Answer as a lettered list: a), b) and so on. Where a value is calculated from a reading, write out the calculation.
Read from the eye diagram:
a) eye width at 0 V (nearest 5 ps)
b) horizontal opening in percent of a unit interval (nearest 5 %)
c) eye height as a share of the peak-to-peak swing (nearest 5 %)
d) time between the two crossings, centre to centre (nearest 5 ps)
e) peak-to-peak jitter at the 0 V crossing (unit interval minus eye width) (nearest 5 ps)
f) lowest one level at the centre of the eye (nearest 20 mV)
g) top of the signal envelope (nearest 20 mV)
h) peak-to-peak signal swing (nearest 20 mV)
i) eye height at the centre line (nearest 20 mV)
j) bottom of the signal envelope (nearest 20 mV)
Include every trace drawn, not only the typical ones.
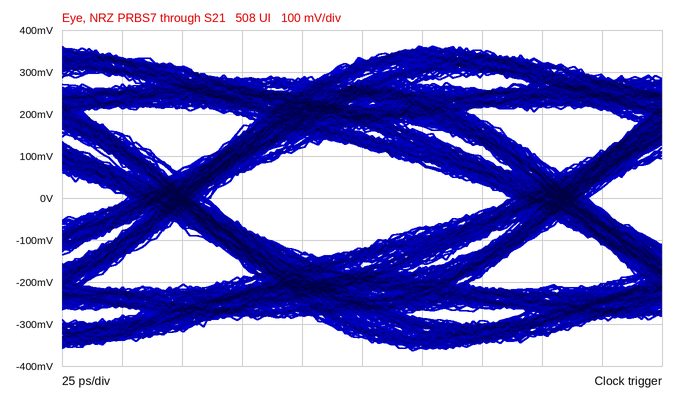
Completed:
a) 125 ps
b) 125 ps / 160 ps ≈ 78.1 %, so 80 % to the nearest 5 %
c) 240 mV / 720 mV ≈ 33.3 %, so 35 % to the nearest 5 %
d) 160 ps
e) 35 ps
f) 120 mV
g) 360 mV
h) 720 mV
i) 240 mV
j) -360 mV
